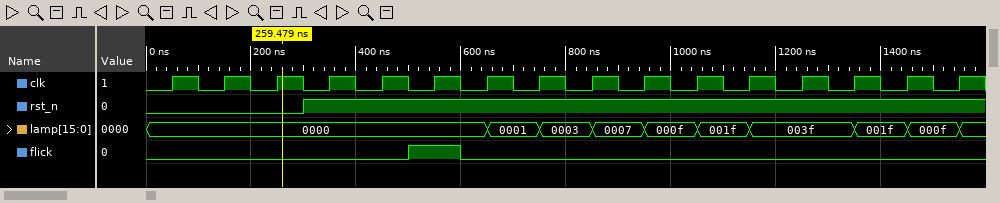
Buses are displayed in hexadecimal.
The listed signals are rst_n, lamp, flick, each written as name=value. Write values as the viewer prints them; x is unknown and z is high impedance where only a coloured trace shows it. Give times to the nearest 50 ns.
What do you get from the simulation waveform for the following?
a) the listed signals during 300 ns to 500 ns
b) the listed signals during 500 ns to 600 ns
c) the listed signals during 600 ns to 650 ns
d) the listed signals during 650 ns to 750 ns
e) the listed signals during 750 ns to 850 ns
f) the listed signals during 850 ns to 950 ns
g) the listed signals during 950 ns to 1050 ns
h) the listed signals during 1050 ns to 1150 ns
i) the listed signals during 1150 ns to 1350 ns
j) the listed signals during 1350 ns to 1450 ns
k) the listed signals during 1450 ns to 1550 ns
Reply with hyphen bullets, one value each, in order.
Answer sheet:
- rst_n=1, lamp=0000, flick=0
- rst_n=1, lamp=0000, flick=1
- rst_n=1, lamp=0000, flick=0
- rst_n=1, lamp=0001, flick=0
- rst_n=1, lamp=0003, flick=0
- rst_n=1, lamp=0007, flick=0
- rst_n=1, lamp=000f, flick=0
- rst_n=1, lamp=001f, flick=0
- rst_n=1, lamp=003f, flick=0
- rst_n=1, lamp=001f, flick=0
- rst_n=1, lamp=000f, flick=0
